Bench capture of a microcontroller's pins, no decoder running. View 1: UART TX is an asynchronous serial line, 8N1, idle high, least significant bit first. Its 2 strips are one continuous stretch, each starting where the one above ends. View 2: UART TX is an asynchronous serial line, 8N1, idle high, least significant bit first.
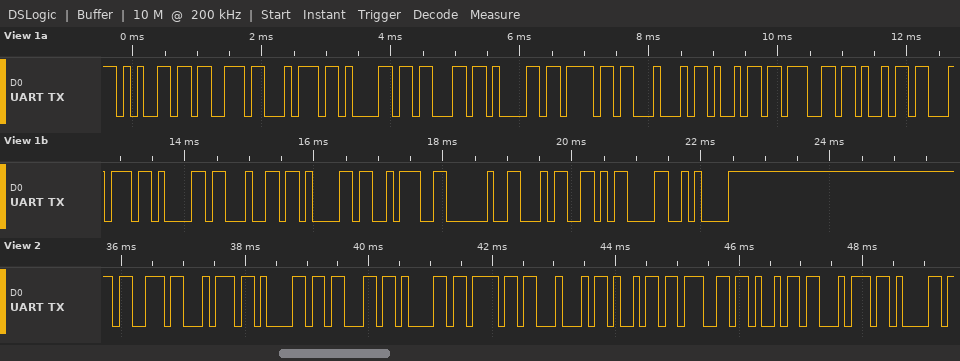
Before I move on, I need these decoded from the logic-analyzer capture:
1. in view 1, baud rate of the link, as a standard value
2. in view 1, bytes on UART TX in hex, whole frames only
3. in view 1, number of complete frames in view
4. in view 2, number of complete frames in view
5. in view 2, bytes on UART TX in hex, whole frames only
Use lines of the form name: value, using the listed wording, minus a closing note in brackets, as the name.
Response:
in view 1, baud rate of the link, as a standard value: 9600 baud
in view 1, bytes on UART TX in hex, whole frames only: 65 73 74 61 63 61 6F 44 69 67 69 74 61 64 61 3A 20 34 0D 0A
in view 1, number of complete frames in view: 20
in view 2, number of complete frames in view: 12
in view 2, bytes on UART TX in hex, whole frames only: 73 74 61 63 61 6F 44 69 67 69 74 61
